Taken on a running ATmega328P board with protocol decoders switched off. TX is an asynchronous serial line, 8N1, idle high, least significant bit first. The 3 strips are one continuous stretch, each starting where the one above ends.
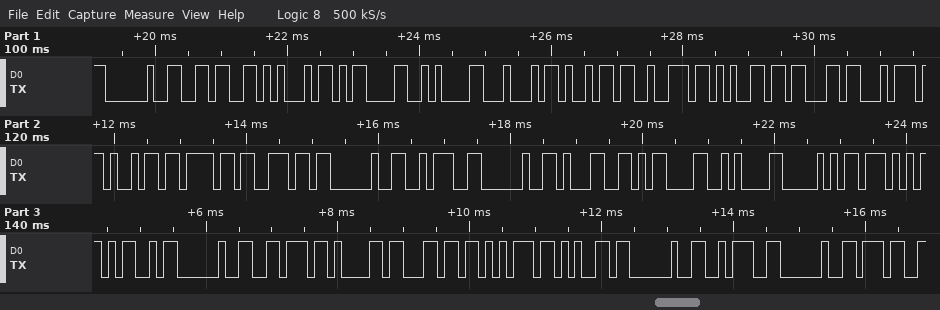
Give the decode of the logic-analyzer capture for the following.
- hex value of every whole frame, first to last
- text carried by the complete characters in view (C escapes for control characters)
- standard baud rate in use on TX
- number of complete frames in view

20 36 45 0D 0A 44 69 72 65 63 74 69 6F 6E 20 3A 20 31 0D 0A 50 57 4D 20 76 61 6C 75 65 20 3A 20 37
" 6E\r\nDirection : 1\r\nPWM value : 7"
9600 baud
33
